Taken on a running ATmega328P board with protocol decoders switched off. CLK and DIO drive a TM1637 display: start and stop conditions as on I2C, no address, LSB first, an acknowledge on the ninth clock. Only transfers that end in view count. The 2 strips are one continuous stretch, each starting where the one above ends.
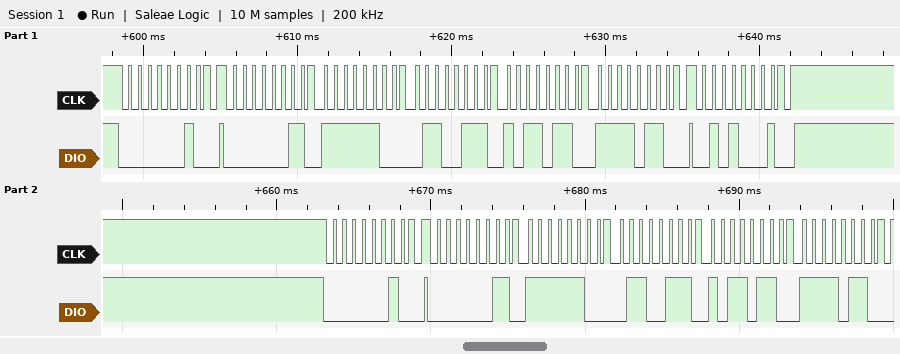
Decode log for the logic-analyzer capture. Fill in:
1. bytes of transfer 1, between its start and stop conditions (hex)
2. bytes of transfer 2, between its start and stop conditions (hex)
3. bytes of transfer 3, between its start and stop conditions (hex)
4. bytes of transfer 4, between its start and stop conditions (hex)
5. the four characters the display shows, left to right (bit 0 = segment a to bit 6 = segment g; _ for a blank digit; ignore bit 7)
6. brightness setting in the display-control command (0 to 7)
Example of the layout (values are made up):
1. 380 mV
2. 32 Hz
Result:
1. 40
2. C0 3F E6 6D 6F
3. 8A
4. 40
5. 0459
6. 2
